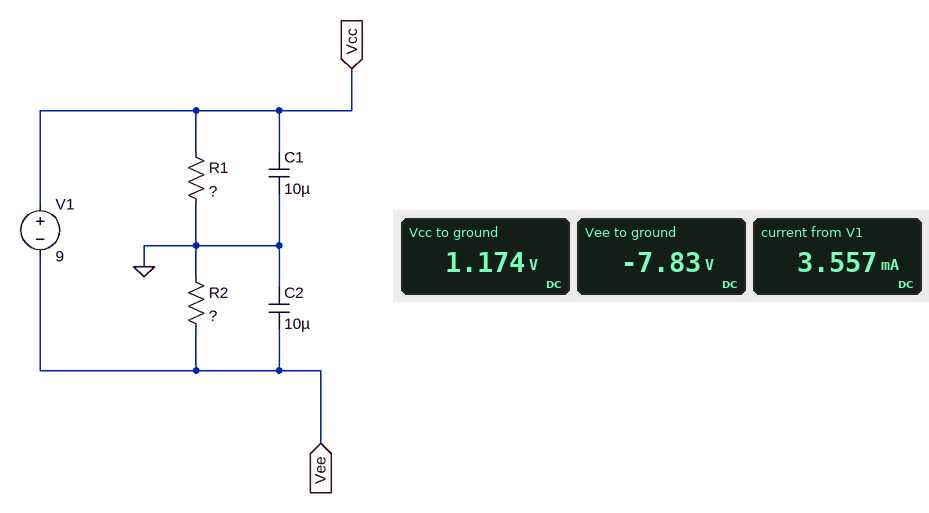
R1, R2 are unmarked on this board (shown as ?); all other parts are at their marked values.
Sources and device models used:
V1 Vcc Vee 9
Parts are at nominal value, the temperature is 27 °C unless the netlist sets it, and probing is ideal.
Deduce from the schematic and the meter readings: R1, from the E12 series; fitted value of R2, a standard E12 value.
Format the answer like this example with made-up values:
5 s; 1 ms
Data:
330 Ω; 2.2 kΩ
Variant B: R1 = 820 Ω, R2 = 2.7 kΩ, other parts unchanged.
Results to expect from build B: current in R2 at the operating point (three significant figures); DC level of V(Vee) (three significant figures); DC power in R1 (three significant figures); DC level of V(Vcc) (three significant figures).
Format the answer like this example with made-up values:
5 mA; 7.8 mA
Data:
2.56 mA; -6.90 V; 5.36 mW; 2.10 V
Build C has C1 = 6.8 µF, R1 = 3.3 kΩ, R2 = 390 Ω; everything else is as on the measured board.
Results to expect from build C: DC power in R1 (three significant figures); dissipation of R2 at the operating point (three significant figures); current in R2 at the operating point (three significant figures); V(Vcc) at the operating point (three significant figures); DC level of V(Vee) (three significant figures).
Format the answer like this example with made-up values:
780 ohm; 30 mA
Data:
19.6 mW; 2.32 mW; 2.44 mA; 8.05 V; -951 mV
